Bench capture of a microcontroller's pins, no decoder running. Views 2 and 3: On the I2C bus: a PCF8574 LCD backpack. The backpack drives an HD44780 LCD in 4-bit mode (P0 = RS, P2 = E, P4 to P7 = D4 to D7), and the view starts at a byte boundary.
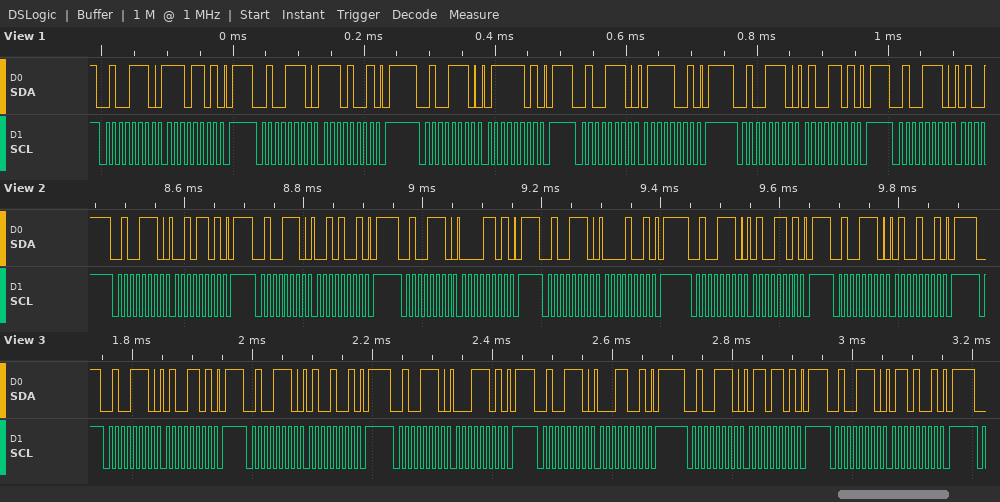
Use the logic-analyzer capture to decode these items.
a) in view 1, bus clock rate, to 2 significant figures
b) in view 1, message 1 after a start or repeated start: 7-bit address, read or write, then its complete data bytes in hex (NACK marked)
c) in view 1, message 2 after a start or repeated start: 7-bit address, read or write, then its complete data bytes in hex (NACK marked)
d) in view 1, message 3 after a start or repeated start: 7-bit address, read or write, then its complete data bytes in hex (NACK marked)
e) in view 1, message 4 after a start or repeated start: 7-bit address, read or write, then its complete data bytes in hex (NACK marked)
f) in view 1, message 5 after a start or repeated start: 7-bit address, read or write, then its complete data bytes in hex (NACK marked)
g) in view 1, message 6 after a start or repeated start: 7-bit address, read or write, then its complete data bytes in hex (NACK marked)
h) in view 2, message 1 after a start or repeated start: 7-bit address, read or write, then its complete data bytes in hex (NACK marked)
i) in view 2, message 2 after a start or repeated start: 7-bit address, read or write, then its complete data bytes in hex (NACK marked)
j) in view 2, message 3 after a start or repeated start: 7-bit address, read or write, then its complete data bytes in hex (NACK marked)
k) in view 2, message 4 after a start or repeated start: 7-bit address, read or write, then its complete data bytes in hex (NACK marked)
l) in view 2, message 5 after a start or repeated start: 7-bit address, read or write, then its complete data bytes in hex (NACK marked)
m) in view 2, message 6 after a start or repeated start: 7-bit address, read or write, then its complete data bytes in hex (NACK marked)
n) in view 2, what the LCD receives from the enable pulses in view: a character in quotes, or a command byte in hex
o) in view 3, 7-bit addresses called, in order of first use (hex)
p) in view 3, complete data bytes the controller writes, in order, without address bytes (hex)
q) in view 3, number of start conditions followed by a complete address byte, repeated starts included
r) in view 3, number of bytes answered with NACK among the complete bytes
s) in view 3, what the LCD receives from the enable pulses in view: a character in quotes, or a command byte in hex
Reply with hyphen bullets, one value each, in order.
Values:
- 100 kHz
- 0x27 write: ED
- 0x27 write: E9
- 0x27 write: 7D
- 0x27 write: 79
- 0x27 write: 4D
- 0x27 write
- 0x27 write: 2D
- 0x27 write: 29
- 0x27 write: 0D
- 0x27 write: 09
- 0x27 write: 4D
- 0x27 write: 49
- ' '
- 0x27
- 4D 49 1D 19 6D 69
- 6
- 0
- 'A'
